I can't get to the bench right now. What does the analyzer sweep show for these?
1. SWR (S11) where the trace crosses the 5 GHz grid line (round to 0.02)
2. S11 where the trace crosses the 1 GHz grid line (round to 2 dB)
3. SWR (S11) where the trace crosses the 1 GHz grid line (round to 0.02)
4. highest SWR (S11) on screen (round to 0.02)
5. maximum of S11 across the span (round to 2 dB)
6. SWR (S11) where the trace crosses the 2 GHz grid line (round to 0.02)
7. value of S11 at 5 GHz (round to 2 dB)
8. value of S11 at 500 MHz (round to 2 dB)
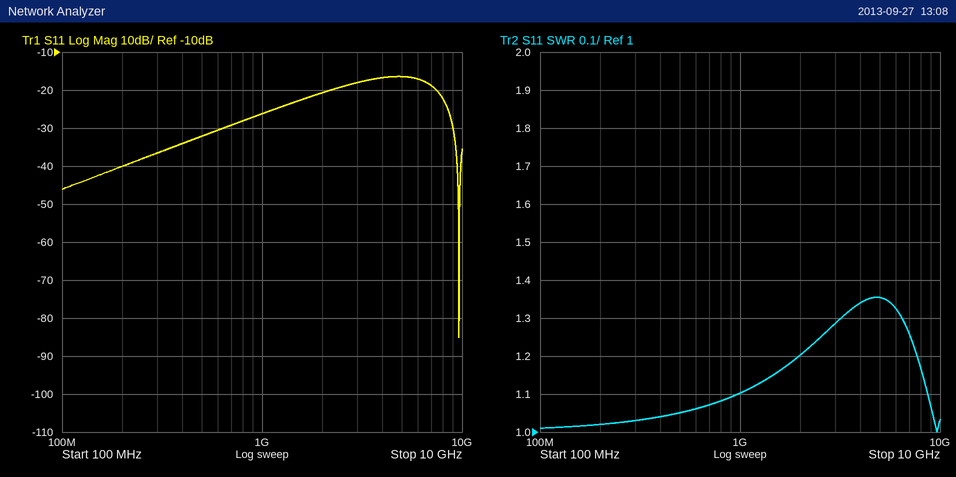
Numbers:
1.36
-26 dB
1.10
1.36
-16 dB
1.20
-16 dB
-32 dB
